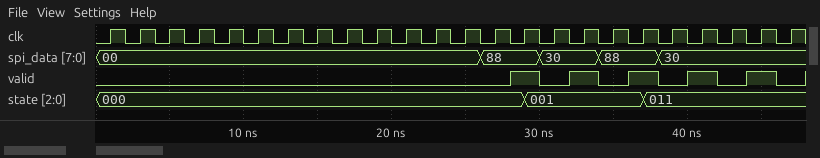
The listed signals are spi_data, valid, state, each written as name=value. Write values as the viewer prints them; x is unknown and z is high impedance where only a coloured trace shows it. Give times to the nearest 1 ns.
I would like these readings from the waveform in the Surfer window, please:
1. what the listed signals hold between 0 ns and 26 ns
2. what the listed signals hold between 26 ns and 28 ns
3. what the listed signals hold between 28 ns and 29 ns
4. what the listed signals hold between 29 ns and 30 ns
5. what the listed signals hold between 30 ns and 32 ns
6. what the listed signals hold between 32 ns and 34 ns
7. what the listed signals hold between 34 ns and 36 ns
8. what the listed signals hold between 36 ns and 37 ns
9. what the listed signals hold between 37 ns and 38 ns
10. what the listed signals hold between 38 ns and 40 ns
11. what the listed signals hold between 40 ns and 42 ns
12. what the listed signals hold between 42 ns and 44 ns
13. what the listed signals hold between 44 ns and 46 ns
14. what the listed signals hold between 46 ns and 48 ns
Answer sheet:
spi_data=00, valid=0, state=000
spi_data=88, valid=0, state=000
spi_data=88, valid=1, state=000
spi_data=88, valid=1, state=001
spi_data=30, valid=0, state=001
spi_data=30, valid=1, state=001
spi_data=88, valid=0, state=001
spi_data=88, valid=1, state=001
spi_data=88, valid=1, state=011
spi_data=30, valid=0, state=011
spi_data=30, valid=1, state=011
spi_data=30, valid=0, state=011
spi_data=30, valid=1, state=011
spi_data=30, valid=0, state=011
